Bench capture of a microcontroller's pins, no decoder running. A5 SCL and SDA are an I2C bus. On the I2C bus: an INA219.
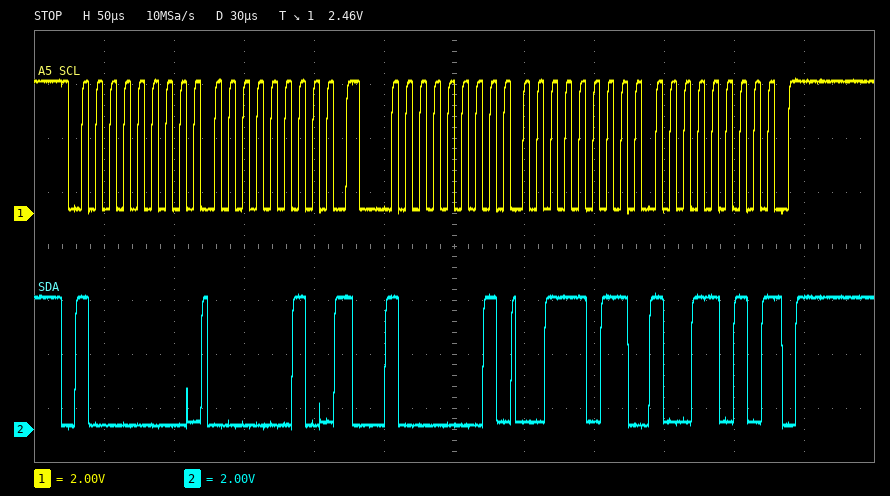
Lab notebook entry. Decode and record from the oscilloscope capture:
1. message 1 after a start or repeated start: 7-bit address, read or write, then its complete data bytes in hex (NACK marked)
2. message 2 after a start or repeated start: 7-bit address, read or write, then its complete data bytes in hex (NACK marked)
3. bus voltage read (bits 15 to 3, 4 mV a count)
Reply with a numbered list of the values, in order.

1. 0x40 write: 02
2. 0x40 read: 3B 9A NACK
3. 7.628 V
